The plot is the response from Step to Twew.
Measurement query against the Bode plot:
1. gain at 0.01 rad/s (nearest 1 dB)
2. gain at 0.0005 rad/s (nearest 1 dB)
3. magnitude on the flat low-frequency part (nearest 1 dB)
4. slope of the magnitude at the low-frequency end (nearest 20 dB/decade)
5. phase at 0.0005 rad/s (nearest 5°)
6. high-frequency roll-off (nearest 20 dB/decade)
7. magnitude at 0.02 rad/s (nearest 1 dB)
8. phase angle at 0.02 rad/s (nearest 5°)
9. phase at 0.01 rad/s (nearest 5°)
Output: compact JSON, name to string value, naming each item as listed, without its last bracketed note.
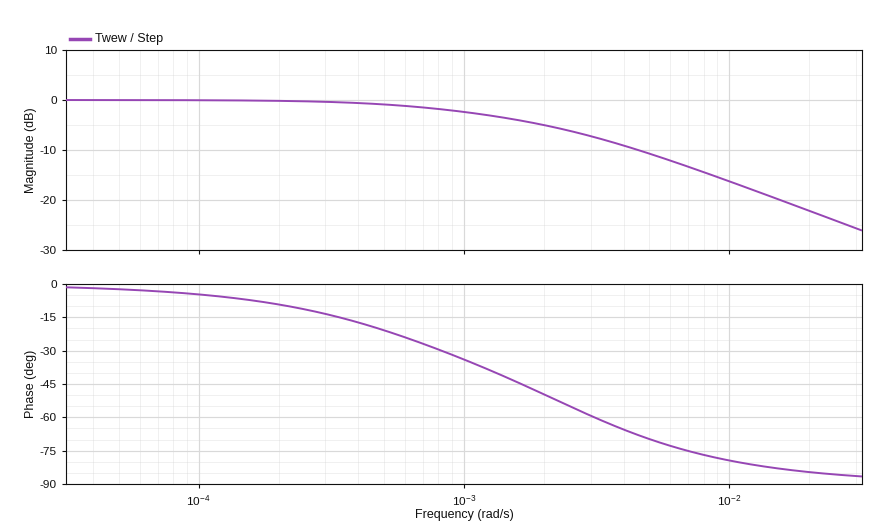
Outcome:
{"gain at 0.01 rad/s": "-16 dB", "gain at 0.0005 rad/s": "-1 dB", "magnitude on the flat low-frequency part": "0 dB", "slope of the magnitude at the low-frequency end": "0 dB/decade", "phase at 0.0005 rad/s": "-20°", "high-frequency roll-off": "-20 dB/decade", "magnitude at 0.02 rad/s": "-22 dB", "phase angle at 0.02 rad/s": "-85°", "phase at 0.01 rad/s": "-80°"}
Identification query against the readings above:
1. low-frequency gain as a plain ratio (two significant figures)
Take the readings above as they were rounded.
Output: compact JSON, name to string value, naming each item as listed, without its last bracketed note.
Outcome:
{"low-frequency gain as a plain ratio": "1.0"}
